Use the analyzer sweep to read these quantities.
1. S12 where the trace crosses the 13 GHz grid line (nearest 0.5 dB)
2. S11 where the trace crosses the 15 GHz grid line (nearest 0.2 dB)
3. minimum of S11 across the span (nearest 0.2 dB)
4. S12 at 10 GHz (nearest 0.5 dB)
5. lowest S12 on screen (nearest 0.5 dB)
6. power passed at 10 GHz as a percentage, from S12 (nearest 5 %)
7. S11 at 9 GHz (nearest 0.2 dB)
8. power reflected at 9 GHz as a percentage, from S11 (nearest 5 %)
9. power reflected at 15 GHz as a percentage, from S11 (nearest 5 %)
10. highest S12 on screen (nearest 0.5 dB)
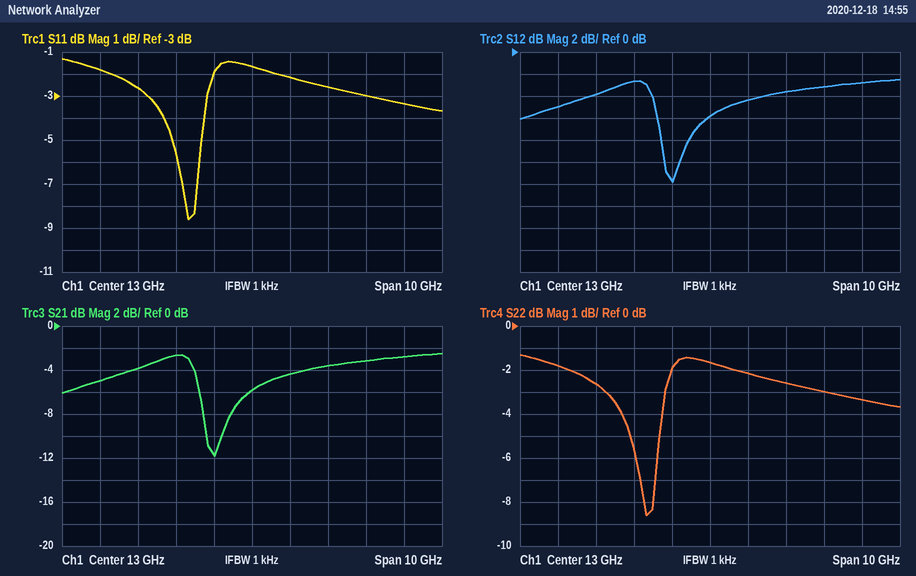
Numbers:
-6.0 dB
-2.6 dB
-8.6 dB
-4.0 dB
-12.0 dB
40 %
-1.8 dB
65 %
55 %
-2.5 dB
